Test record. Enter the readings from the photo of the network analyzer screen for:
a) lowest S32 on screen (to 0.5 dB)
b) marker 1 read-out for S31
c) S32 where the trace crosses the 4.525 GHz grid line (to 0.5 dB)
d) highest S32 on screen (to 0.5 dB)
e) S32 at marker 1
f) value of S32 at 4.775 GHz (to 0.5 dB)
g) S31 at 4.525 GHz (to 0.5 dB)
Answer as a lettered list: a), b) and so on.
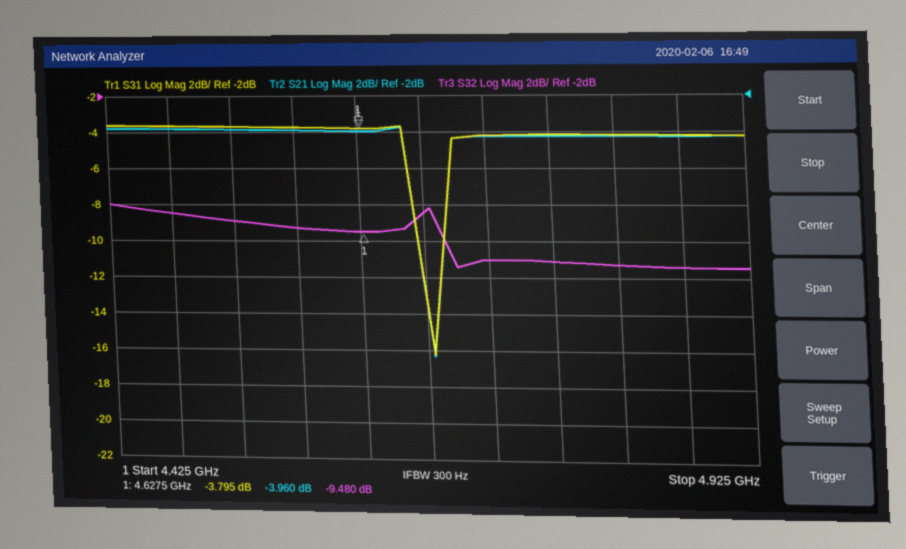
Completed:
a) -11.5 dB
b) -3.795 dB
c) -9.0 dB
d) -8.0 dB
e) -9.480 dB
f) -11.0 dB
g) -3.5 dB
